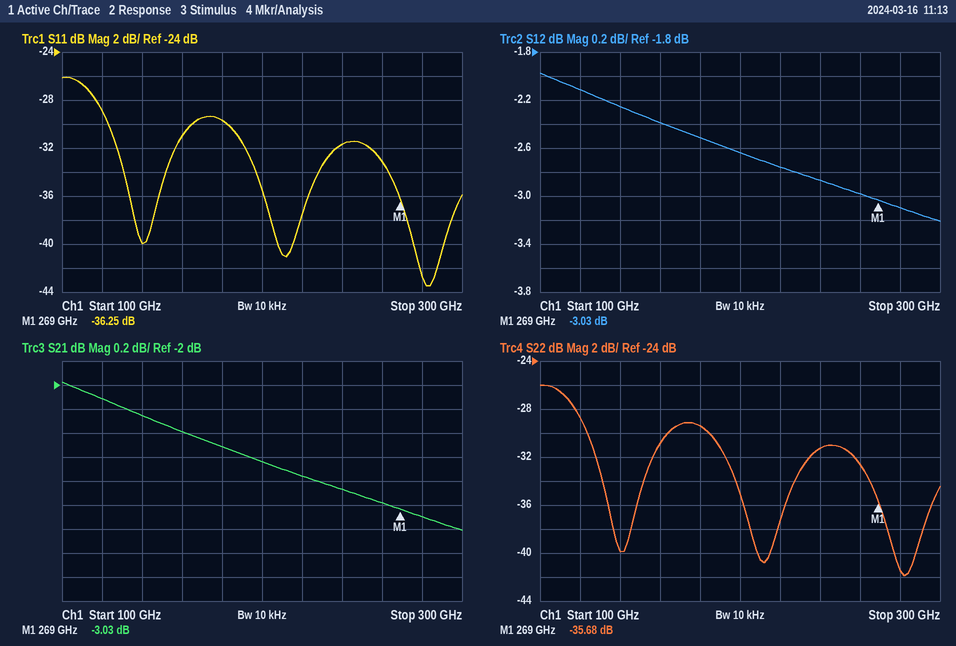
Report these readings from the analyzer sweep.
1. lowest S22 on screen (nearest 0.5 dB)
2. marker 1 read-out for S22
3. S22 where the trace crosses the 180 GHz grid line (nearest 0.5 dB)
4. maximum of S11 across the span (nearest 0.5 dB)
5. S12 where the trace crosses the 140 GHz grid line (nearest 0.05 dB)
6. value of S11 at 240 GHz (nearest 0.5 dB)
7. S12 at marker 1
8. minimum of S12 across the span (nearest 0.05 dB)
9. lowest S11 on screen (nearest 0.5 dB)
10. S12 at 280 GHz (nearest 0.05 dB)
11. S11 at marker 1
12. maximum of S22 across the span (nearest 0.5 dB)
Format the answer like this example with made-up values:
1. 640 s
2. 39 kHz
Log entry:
1. -42.0 dB
2. -35.68 dB
3. -29.5 dB
4. -26.0 dB
5. -2.25 dB
6. -31.5 dB
7. -3.03 dB
8. -3.20 dB
9. -43.5 dB
10. -3.10 dB
11. -36.25 dB
12. -26.0 dB
